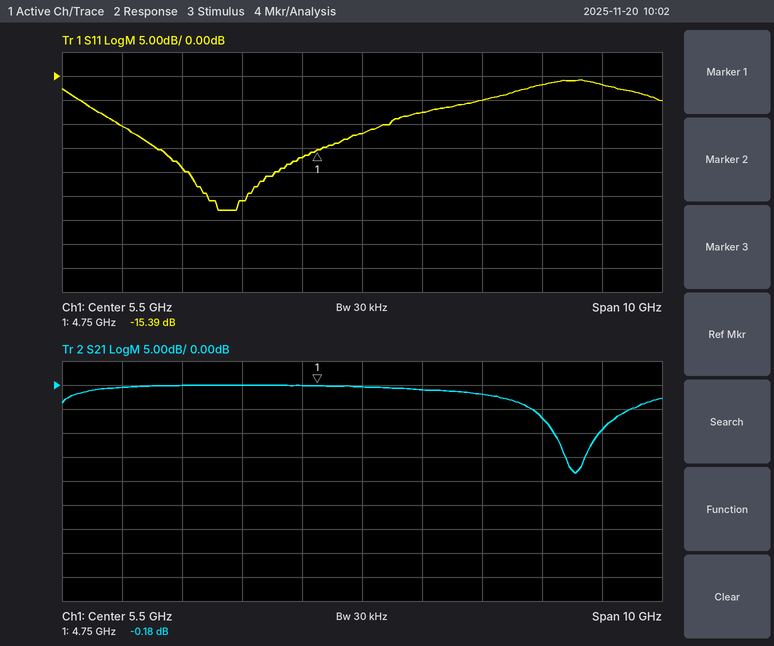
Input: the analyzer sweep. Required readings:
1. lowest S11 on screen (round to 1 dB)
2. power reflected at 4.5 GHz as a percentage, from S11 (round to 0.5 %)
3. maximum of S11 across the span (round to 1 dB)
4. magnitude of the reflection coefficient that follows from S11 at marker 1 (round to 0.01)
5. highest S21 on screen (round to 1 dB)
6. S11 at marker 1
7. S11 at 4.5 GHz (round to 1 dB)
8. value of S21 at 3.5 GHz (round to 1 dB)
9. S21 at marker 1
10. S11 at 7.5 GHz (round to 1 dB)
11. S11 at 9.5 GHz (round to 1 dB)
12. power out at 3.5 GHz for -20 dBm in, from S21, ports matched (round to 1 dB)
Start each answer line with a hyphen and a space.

- -28 dB
- 2.0 %
- -1 dB
- 0.17
- 0 dB
- -15.39 dB
- -17 dB
- 0 dB
- -0.18 dB
- -5 dB
- -2 dB
- -20 dBm
